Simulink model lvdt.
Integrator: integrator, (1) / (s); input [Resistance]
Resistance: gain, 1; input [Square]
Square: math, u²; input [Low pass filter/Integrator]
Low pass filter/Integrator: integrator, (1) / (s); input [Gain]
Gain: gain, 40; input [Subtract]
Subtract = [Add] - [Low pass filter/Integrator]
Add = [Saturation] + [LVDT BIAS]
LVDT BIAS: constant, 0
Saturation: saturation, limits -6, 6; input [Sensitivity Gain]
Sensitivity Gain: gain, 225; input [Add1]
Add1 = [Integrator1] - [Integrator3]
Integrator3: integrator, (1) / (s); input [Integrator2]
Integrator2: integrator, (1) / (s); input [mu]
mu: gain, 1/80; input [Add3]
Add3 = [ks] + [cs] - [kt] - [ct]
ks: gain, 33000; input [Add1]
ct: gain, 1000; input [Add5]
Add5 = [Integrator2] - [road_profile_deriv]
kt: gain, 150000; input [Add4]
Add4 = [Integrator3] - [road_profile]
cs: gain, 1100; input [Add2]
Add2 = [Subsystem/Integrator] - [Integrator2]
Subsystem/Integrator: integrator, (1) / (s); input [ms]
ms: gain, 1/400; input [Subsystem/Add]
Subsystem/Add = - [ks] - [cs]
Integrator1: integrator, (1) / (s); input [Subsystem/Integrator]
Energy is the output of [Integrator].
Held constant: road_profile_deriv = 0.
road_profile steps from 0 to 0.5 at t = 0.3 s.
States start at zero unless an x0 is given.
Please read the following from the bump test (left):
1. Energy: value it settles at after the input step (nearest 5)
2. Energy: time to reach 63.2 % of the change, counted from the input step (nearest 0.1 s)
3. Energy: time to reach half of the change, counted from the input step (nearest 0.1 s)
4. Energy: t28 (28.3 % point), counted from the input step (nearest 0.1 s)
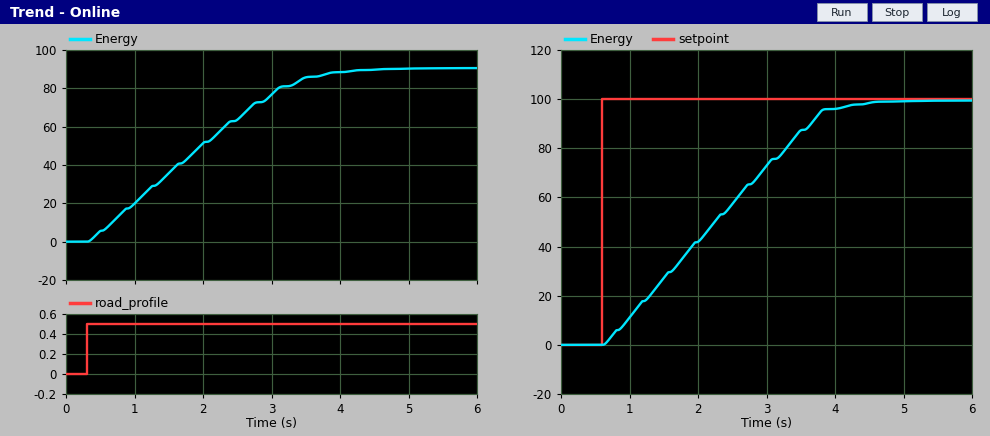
90
1.9 s
1.5 s
0.9 s
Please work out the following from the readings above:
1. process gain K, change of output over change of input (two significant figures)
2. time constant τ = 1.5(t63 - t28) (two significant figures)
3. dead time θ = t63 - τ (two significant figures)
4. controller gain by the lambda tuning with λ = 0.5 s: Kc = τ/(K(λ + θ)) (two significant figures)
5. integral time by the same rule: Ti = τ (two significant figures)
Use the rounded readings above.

180
1.5 s
0.40 s
0.0093
1.5 s
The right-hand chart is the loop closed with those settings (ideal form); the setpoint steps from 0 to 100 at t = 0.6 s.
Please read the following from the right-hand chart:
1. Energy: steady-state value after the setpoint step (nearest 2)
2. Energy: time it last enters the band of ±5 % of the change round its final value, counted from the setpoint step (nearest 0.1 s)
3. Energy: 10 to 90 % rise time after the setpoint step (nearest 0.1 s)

100
3.2 s
2.7 s
